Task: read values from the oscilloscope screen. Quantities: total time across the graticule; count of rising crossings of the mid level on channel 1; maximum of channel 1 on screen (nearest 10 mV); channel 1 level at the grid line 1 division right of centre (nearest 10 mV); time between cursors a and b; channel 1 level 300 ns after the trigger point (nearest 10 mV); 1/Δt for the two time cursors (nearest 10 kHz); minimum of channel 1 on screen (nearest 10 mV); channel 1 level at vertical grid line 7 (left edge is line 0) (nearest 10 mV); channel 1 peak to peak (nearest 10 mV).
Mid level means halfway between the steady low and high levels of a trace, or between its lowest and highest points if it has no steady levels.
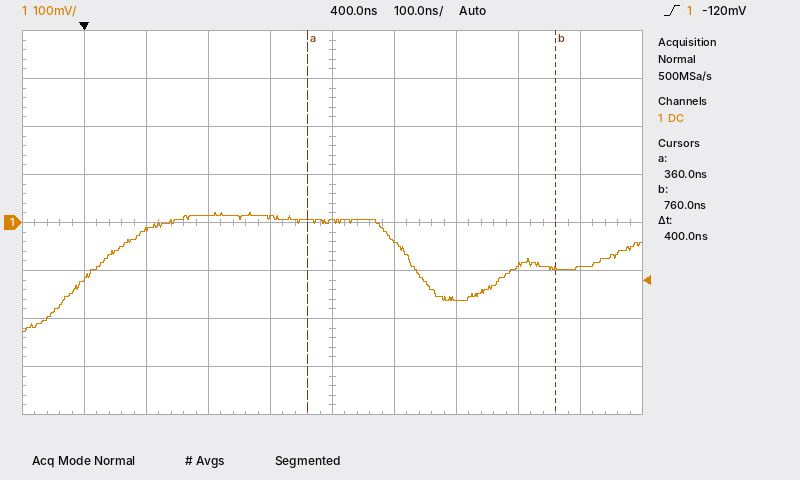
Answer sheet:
1 µs
2
20 mV
-40 mV
400 ns
10 mV
2.50 MHz
-230 mV
-160 mV
250 mV
